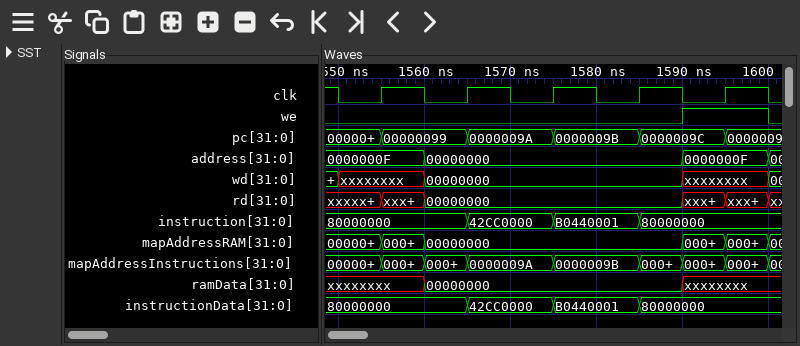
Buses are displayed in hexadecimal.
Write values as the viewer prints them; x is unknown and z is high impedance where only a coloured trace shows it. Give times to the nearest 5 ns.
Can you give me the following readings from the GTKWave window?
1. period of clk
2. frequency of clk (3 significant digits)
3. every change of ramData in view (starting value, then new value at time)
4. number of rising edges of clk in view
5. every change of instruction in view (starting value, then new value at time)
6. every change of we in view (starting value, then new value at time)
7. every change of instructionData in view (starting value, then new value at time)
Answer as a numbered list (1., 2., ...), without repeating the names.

1. 10 ns
2. 100 MHz
3. xxxxxxxx, 00000000 at 1560 ns, xxxxxxxx at 1590 ns
4. 5
5. 80000000, 42CC0000 at 1565 ns, B0440001 at 1575 ns, 80000000 at 1585 ns
6. 0, 1 at 1590 ns, 0 at 1600 ns
7. 80000000, 42CC0000 at 1565 ns, B0440001 at 1575 ns, 80000000 at 1585 ns
